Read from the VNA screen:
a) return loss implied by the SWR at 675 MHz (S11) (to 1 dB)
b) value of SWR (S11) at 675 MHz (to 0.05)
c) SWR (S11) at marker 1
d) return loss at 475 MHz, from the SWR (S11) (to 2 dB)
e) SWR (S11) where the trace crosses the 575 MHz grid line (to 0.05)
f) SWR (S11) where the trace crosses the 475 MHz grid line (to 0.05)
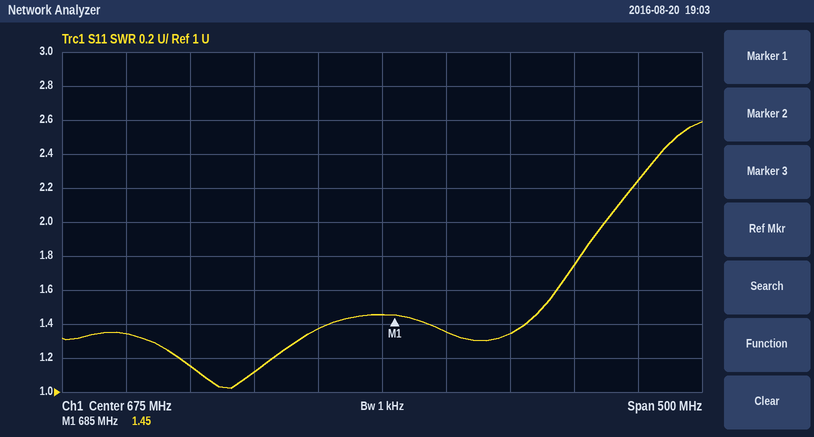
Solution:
15 dB
1.45
1.45
16 dB
1.10
1.35
